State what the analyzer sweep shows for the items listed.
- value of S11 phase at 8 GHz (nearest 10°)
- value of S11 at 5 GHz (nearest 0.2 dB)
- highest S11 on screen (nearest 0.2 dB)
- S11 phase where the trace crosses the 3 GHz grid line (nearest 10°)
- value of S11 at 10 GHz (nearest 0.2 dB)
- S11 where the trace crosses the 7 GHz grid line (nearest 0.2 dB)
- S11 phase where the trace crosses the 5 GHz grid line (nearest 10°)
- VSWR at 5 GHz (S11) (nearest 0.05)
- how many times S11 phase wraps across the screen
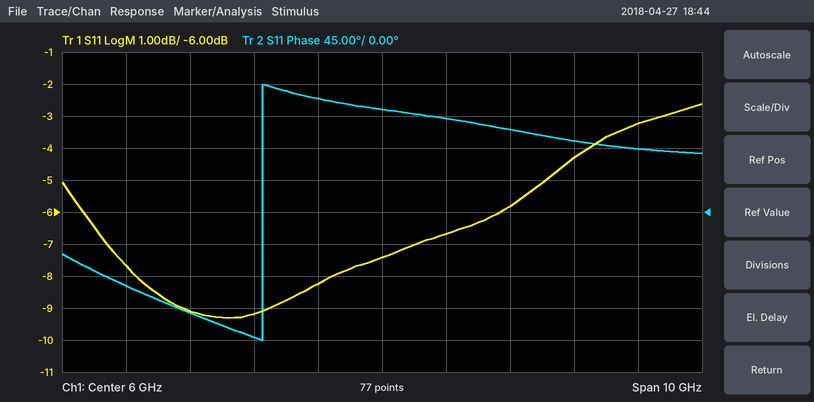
120°
-8.2 dB
-2.6 dB
-140°
-3.2 dB
-6.6 dB
160°
2.25
1
